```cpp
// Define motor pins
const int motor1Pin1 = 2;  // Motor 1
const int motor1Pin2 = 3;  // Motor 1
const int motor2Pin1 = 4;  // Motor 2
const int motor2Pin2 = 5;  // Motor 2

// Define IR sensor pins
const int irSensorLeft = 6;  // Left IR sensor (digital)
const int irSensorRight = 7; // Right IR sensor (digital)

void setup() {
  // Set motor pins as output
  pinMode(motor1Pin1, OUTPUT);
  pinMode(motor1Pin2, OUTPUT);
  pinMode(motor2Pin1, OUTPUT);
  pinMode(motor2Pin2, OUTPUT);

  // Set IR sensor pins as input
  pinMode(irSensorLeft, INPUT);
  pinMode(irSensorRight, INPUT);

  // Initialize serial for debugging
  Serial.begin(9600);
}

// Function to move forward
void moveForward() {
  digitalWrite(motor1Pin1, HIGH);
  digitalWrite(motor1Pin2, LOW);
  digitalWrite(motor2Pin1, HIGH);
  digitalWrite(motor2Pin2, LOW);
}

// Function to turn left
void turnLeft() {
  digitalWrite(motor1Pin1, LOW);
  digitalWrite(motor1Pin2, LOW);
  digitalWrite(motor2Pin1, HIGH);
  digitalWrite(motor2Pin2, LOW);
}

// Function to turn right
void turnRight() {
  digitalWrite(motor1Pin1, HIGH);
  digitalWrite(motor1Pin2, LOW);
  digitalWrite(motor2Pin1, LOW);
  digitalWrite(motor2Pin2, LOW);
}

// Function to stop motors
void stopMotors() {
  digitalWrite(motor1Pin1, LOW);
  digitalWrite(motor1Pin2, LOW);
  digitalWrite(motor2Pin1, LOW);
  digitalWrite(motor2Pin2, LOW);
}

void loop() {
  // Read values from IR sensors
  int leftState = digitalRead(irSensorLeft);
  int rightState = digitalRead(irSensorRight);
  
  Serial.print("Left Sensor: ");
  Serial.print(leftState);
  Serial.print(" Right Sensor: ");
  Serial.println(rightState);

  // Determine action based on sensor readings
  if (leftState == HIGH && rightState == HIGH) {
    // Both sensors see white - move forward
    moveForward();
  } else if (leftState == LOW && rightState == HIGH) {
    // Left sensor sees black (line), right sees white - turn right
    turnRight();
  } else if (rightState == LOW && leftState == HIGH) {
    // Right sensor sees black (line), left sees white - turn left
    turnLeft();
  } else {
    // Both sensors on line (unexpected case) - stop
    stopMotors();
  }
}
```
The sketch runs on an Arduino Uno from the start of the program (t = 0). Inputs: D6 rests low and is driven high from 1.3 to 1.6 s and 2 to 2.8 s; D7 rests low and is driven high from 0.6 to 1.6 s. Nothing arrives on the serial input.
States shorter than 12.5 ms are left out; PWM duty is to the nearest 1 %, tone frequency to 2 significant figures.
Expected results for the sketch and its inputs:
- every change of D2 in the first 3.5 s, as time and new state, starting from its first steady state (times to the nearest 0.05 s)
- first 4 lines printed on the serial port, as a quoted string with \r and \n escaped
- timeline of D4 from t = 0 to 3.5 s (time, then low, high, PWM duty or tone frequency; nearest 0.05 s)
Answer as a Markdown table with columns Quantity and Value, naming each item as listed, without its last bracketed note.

| Quantity | Value |
|---|---|
| every change of D2 in the first 3.5 s, as time and new state, starting from its first steady state | 0 s low; 0.65 s high; 1.65 s low |
| first 4 lines printed on the serial port, as a quoted string with \r and \n escaped | "Left Sensor: 0 Right Sensor: 0\r\nLeft Sensor: 0 Right Sensor: 0\r\nLeft Sensor: 0 Right Sensor: 0\r\nLeft Sensor: 0 Right Sensor: 0\r\n" |
| timeline of D4 from t = 0 to 3.5 s | 0 s low; 1.35 s high; 1.65 s low; 2.05 s high; 2.85 s low |
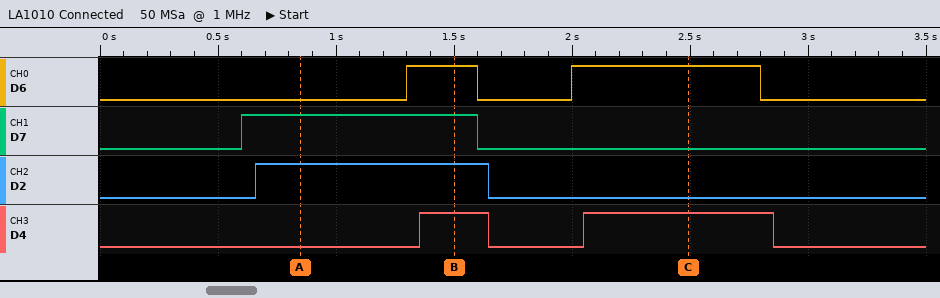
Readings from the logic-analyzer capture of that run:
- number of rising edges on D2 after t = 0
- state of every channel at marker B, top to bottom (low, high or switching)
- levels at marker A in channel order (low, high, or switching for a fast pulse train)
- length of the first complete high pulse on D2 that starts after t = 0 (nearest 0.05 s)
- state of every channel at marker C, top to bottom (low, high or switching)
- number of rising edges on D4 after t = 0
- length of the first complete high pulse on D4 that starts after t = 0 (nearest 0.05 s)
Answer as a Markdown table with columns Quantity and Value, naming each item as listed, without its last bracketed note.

| Quantity | Value |
|---|---|
| number of rising edges on D2 after t = 0 | 1 |
| state of every channel at marker B, top to bottom | D6 high, D7 high, D2 high, D4 high |
| levels at marker A in channel order | D6 low, D7 high, D2 high, D4 low |
| length of the first complete high pulse on D2 that starts after t = 0 | 1.00 s |
| state of every channel at marker C, top to bottom | D6 high, D7 low, D2 low, D4 high |
| number of rising edges on D4 after t = 0 | 2 |
| length of the first complete high pulse on D4 that starts after t = 0 | 0.30 s |
